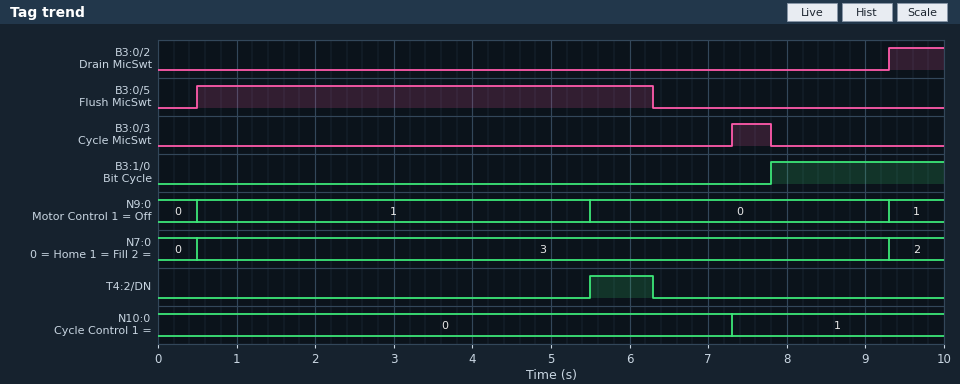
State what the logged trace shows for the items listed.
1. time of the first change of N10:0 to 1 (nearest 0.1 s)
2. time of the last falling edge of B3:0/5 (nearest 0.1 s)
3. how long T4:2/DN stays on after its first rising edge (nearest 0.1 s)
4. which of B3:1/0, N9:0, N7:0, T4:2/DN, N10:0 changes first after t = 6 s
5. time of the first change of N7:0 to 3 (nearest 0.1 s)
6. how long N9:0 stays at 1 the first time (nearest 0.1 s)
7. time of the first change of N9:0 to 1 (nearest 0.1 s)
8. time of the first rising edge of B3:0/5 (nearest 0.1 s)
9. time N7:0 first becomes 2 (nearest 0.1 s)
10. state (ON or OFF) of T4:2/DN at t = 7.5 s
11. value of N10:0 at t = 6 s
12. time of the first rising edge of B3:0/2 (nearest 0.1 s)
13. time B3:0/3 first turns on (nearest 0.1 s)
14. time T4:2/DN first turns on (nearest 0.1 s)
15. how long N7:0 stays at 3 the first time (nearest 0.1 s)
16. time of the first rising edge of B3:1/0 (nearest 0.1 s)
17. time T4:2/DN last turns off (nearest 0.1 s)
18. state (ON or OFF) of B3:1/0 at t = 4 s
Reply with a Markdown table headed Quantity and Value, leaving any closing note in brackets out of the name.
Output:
| Quantity | Value |
|---|---|
| time of the first change of N10:0 to 1 | 7.3 s |
| time of the last falling edge of B3:0/5 | 6.3 s |
| how long T4:2/DN stays on after its first rising edge | 0.8 s |
| which of B3:1/0, N9:0, N7:0, T4:2/DN, N10:0 changes first after t = 6 s | T4:2/DN |
| time of the first change of N7:0 to 3 | 0.5 s |
| how long N9:0 stays at 1 the first time | 5.0 s |
| time of the first change of N9:0 to 1 | 0.5 s |
| time of the first rising edge of B3:0/5 | 0.5 s |
| time N7:0 first becomes 2 | 9.3 s |
| state (ON or OFF) of T4:2/DN at t = 7.5 s | OFF |
| value of N10:0 at t = 6 s | 0 |
| time of the first rising edge of B3:0/2 | 9.3 s |
| time B3:0/3 first turns on | 7.3 s |
| time T4:2/DN first turns on | 5.5 s |
| how long N7:0 stays at 3 the first time | 8.8 s |
| time of the first rising edge of B3:1/0 | 7.8 s |
| time T4:2/DN last turns off | 6.3 s |
| state (ON or OFF) of B3:1/0 at t = 4 s | OFF |
